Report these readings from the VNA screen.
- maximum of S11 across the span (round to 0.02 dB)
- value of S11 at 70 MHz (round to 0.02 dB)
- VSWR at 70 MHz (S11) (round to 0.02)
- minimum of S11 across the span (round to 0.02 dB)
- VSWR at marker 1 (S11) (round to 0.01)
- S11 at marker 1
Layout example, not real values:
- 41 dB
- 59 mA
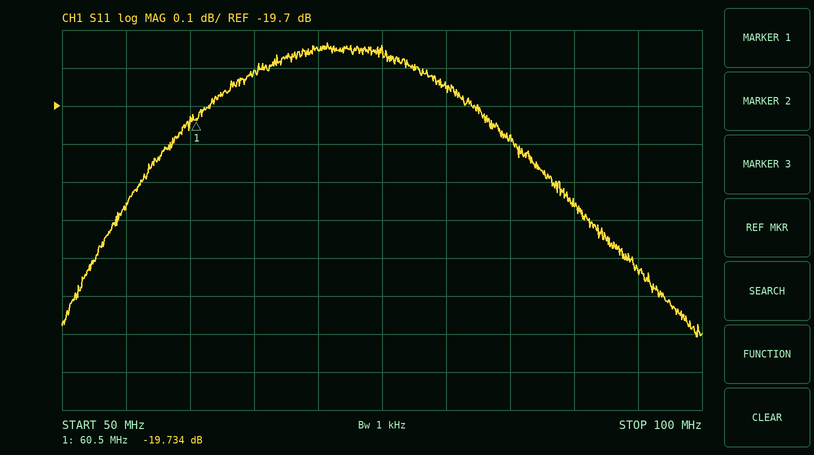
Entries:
- -19.54 dB
- -19.56 dB
- 1.24
- -20.30 dB
- 1.23
- -19.734 dB
